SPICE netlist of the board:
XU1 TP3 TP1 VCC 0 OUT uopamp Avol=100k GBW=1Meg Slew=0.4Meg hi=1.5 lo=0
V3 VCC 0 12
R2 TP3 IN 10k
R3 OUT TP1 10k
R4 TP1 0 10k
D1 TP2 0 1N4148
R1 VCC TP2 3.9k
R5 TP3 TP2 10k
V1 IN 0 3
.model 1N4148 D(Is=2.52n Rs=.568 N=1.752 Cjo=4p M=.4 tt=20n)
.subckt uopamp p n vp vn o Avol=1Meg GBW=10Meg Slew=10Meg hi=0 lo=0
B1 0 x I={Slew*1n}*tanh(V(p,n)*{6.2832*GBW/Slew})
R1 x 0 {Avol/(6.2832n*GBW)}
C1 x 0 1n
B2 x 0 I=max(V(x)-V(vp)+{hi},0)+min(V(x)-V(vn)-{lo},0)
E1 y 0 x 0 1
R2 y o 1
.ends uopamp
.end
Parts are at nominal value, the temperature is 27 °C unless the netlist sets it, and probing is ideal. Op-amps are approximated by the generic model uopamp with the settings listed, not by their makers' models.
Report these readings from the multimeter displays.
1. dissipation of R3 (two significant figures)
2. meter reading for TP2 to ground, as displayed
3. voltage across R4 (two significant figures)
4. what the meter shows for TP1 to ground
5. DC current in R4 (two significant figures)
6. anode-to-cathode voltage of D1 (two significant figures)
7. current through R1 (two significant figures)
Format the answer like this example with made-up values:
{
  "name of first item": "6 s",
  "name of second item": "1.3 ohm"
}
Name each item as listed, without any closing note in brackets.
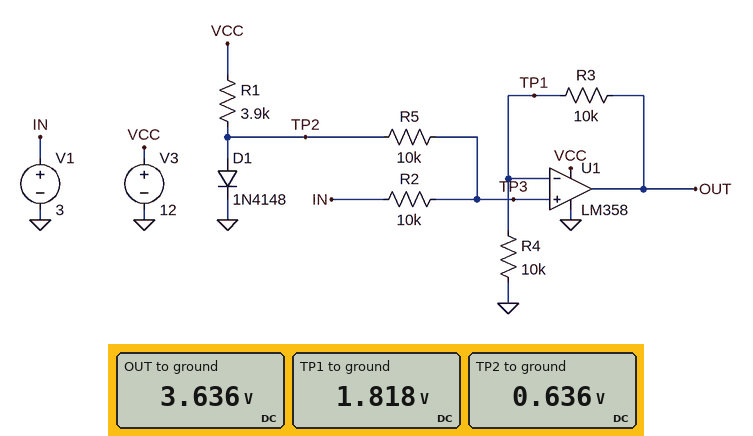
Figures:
{
  "dissipation of R3": "330 µW",
  "meter reading for TP2 to ground, as displayed": "0.636 V",
  "voltage across R4": "1.8 V",
  "what the meter shows for TP1 to ground": "1.818 V",
  "DC current in R4": "180 µA",
  "anode-to-cathode voltage of D1": "640 mV",
  "current through R1": "2.9 mA"
}
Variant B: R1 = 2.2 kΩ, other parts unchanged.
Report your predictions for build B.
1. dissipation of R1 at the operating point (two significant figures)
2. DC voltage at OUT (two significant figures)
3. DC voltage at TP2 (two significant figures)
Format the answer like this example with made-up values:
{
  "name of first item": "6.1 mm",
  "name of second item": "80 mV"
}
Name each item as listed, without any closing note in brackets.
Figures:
{
  "dissipation of R1 at the operating point": "58 mW",
  "DC voltage at OUT": "3.7 V",
  "DC voltage at TP2": "660 mV"
}
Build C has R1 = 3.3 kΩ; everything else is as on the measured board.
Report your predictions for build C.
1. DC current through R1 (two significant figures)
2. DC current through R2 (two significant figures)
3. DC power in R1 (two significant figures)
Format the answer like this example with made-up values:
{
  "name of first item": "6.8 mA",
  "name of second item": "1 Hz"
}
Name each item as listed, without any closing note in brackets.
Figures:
{
  "DC current through R1": "3.4 mA",
  "DC current through R2": "120 µA",
  "DC power in R1": "39 mW"
}
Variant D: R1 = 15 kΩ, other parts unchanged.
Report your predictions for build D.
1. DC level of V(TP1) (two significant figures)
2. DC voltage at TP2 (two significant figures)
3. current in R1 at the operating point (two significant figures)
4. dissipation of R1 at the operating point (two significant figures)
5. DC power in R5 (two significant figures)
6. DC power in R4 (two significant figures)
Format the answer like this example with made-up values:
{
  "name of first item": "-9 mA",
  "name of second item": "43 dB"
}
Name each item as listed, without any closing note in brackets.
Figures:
{
  "DC level of V(TP1)": "1.8 V",
  "DC voltage at TP2": "580 mV",
  "current in R1 at the operating point": "760 µA",
  "dissipation of R1 at the operating point": "8.7 mW",
  "DC power in R5": "150 µW",
  "DC power in R4": "320 µW"
}
